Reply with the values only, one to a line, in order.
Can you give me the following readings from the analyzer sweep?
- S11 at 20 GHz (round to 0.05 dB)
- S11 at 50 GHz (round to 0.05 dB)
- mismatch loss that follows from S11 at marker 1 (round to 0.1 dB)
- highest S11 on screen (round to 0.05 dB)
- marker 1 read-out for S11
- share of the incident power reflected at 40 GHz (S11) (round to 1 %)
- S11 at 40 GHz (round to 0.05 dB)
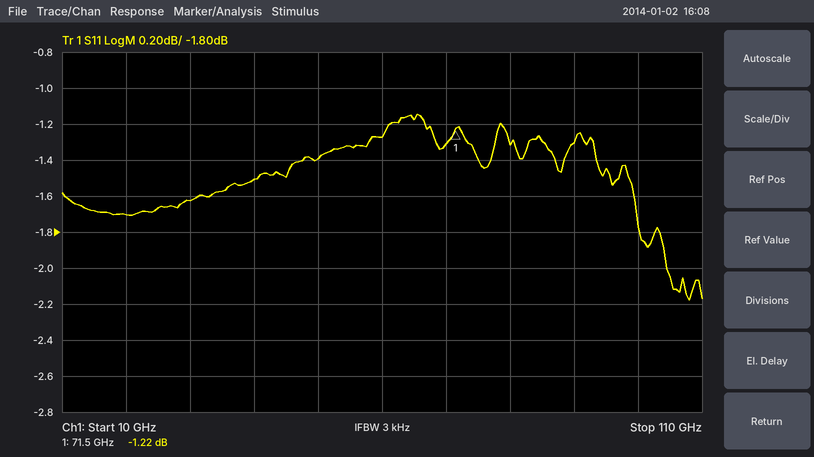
-1.70 dB
-1.40 dB
6.1 dB
-1.15 dB
-1.22 dB
71 %
-1.50 dB
